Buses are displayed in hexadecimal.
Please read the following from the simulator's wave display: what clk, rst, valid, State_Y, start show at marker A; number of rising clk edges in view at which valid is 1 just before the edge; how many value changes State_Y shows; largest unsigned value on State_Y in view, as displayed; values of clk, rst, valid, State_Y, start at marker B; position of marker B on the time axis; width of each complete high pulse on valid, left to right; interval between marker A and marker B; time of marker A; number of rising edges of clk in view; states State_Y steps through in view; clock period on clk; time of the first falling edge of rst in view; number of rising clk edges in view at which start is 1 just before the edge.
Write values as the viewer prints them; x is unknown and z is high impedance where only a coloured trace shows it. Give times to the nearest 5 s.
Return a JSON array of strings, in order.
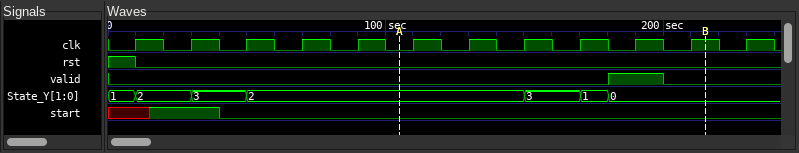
["clk=0, rst=0, valid=0, State_Y=2, start=0", "1", "6", "3", "clk=1, rst=0, valid=0, State_Y=0, start=0", "215 s", "20 s", "110 s", "105 s", "12", "1, 2, 3, 2, 3, 1, 0", "20 s", "10 s", "1"]
